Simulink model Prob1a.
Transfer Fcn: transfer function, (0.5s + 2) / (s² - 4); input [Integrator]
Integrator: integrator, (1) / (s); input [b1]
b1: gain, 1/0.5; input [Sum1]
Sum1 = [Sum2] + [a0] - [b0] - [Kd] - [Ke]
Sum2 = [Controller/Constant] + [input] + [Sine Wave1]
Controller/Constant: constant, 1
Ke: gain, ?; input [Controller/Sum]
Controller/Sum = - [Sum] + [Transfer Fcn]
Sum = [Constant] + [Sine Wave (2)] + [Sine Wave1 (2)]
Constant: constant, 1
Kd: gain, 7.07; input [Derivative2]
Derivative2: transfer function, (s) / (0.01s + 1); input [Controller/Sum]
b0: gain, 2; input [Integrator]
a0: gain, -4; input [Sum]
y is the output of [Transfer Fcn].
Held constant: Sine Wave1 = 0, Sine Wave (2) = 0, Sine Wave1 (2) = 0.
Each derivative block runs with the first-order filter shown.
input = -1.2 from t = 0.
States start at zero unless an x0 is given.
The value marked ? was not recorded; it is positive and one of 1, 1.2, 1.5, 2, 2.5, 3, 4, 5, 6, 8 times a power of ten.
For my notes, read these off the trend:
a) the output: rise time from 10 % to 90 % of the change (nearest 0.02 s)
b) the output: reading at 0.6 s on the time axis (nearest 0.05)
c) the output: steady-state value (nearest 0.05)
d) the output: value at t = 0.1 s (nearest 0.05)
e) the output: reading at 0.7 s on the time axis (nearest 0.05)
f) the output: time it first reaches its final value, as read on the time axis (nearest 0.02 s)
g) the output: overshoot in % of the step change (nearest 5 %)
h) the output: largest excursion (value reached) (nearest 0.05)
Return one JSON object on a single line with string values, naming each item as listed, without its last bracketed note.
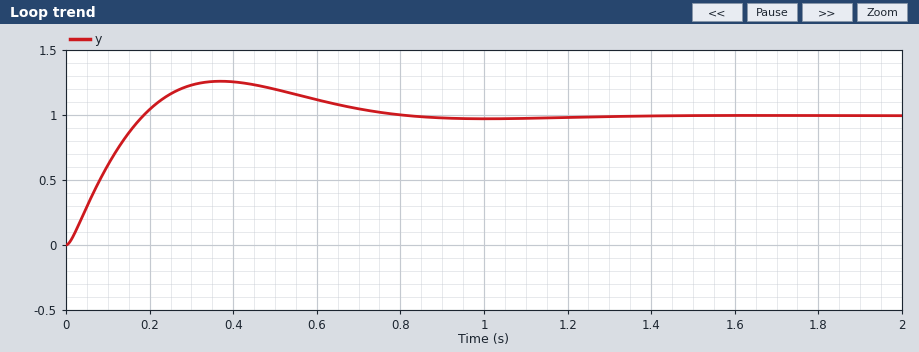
{"the output: rise time from 10 % to 90 % of the change": "0.14 s", "the output: reading at 0.6 s on the time axis": "1.10", "the output: steady-state value": "1.00", "the output: value at t = 0.1 s": "0.60", "the output: reading at 0.7 s on the time axis": "1.05", "the output: time it first reaches its final value, as read on the time axis": "0.18 s", "the output: overshoot in % of the step change": "25 %", "the output: largest excursion (value reached)": "1.25"}
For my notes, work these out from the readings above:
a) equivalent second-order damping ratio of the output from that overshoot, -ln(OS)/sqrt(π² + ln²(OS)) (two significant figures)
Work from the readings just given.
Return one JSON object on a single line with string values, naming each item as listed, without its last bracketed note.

{"equivalent second-order damping ratio of the output from that overshoot, -ln(OS)/sqrt(π² + ln²(OS))": "0.40"}
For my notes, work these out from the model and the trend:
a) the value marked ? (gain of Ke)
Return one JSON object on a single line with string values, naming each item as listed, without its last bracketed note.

{"the value marked ?": "40"}
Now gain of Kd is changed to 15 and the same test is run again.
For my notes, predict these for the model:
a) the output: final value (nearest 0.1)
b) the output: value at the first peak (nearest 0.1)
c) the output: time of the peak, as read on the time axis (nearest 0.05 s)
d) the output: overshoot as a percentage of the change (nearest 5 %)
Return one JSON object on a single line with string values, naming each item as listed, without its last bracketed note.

{"the output: final value": "1.0", "the output: value at the first peak": "1.1", "the output: time of the peak, as read on the time axis": "0.25 s", "the output: overshoot as a percentage of the change": "10 %"}
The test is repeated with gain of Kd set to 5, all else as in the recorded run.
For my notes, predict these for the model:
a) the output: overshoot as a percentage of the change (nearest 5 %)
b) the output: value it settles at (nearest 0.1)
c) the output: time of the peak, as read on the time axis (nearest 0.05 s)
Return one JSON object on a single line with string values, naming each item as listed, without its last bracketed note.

{"the output: overshoot as a percentage of the change": "35 %", "the output: value it settles at": "1.0", "the output: time of the peak, as read on the time axis": "0.40 s"}
